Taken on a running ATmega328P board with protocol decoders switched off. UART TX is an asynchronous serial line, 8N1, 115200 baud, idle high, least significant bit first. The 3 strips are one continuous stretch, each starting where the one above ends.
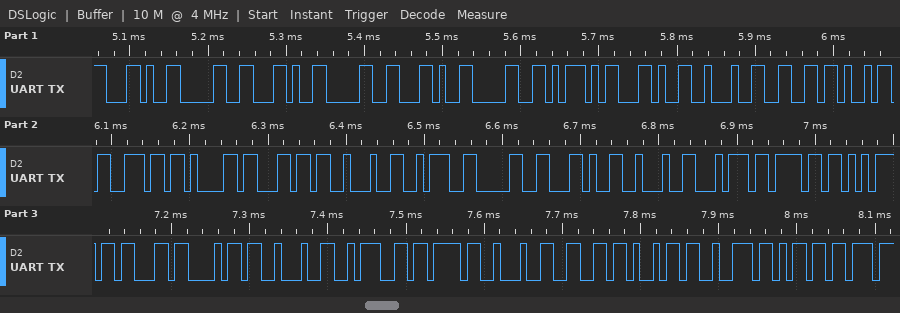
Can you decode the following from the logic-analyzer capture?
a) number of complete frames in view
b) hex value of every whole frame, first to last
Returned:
32
2C 30 2C 30 2C 30 5D 2C 22 66 69 6E 61 6C 22 3A 30 2C 22 74 6F 75 63 68 22 3A 7B 22 66 69 72 6D
